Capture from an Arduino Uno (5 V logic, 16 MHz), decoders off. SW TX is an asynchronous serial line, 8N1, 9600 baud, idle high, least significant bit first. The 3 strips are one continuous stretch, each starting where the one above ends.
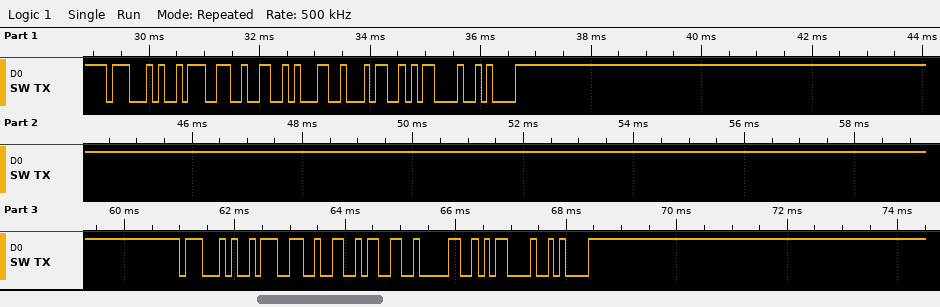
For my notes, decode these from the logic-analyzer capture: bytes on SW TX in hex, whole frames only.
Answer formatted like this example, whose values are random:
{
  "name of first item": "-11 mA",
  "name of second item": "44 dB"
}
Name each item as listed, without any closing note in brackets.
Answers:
{
  "bytes on SW TX in hex, whole frames only": "0x47 0x3A 0x32 0x31 0x34 0x0D 0x0A 0x47 0x3A 0x32 0x33 0x30 0x0D 0x0A"
}
